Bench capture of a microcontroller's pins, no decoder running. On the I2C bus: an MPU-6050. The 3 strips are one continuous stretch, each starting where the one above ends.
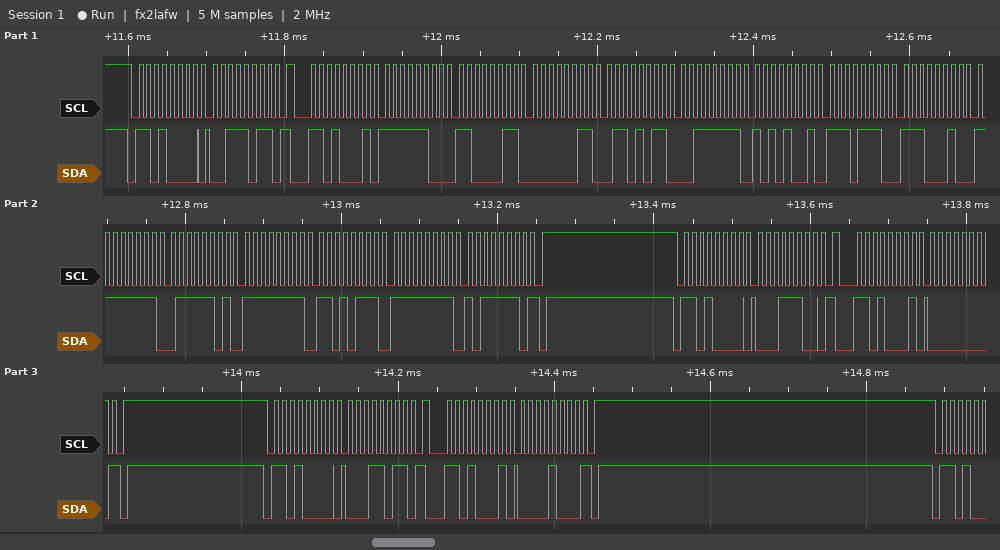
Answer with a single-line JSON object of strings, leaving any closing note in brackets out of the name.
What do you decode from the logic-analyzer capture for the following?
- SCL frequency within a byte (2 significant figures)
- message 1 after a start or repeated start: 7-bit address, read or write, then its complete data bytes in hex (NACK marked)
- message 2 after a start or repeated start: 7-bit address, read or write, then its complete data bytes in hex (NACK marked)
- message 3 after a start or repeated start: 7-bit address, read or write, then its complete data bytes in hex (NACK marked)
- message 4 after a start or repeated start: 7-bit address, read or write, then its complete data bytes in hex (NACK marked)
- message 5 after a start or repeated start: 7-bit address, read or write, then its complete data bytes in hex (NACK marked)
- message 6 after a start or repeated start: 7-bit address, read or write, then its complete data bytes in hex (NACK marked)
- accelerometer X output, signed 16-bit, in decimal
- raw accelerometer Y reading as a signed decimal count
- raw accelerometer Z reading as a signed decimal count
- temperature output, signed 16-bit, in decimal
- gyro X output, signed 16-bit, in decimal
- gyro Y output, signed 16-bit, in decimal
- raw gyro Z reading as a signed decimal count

{"SCL frequency within a byte": "100 kHz", "message 1 after a start or repeated start: 7-bit address, read or write, then its complete data bytes in hex": "0x68 write: 3B", "message 2 after a start or repeated start: 7-bit address, read or write, then its complete data bytes in hex": "0x68 read: FC C3 03 6B 3F A9 EE E2 FF 7D FF D7 FF BE NACK", "message 3 after a start or repeated start: 7-bit address, read or write, then its complete data bytes in hex": "0x68 write: 1C", "message 4 after a start or repeated start: 7-bit address, read or write, then its complete data bytes in hex": "0x68 read: 00 NACK", "message 5 after a start or repeated start: 7-bit address, read or write, then its complete data bytes in hex": "0x68 write: 1B", "message 6 after a start or repeated start: 7-bit address, read or write, then its complete data bytes in hex": "0x68 read: 08 NACK", "accelerometer X output, signed 16-bit, in decimal": "-829", "raw accelerometer Y reading as a signed decimal count": "875", "raw accelerometer Z reading as a signed decimal count": "16297", "temperature output, signed 16-bit, in decimal": "-4382", "gyro X output, signed 16-bit, in decimal": "-131", "gyro Y output, signed 16-bit, in decimal": "-41", "raw gyro Z reading as a signed decimal count": "-66"}
